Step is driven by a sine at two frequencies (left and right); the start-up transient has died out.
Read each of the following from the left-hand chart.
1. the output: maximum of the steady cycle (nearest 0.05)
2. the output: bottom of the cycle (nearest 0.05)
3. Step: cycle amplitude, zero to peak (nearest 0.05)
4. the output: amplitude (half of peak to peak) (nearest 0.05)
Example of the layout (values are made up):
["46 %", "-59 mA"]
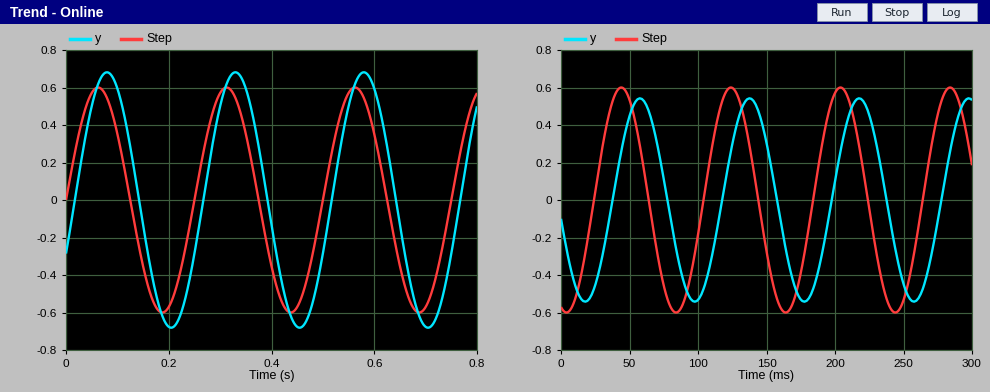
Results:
["0.70", "-0.70", "0.60", "0.70"]
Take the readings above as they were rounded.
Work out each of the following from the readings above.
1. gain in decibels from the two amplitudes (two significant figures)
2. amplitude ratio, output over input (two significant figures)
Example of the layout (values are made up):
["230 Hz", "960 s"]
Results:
["1.3 dB", "1.2"]
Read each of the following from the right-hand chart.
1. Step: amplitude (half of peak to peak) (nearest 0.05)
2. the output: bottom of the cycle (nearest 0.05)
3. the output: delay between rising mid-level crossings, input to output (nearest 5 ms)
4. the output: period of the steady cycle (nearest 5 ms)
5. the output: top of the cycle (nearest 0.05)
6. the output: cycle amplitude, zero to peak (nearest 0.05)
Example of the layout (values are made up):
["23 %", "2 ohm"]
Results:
["0.60", "-0.55", "15 ms", "80 ms", "0.55", "0.55"]
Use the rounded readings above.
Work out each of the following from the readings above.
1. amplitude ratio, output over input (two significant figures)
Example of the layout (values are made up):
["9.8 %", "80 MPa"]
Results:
["0.92"]
